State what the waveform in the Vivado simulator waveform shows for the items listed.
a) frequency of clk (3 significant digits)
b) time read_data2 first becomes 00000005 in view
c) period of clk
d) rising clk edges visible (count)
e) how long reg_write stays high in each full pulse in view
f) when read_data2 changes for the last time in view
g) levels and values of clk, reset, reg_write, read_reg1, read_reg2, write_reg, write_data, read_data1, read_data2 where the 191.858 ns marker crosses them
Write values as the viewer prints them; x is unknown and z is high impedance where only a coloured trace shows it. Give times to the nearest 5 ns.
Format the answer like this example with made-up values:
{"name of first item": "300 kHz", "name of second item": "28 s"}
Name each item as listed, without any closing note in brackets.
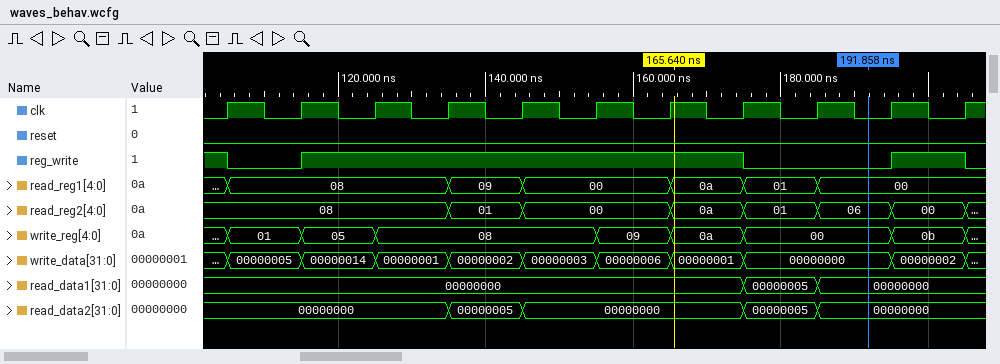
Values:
{"frequency of clk": "100 MHz", "time read_data2 first becomes 00000005 in view": "135 ns", "period of clk": "10 ns", "rising clk edges visible": "11", "how long reg_write stays high in each full pulse in view": "60 ns, 10 ns", "when read_data2 changes for the last time in view": "185 ns", "levels and values of clk, reset, reg_write, read_reg1, read_reg2, write_reg, write_data, read_data1, read_data2 where the 191.858 ns marker crosses them": "clk=0, reset=0, reg_write=0, read_reg1=00, read_reg2=06, write_reg=00, write_data=00000000, read_data1=00000000, read_data2=00000000"}
